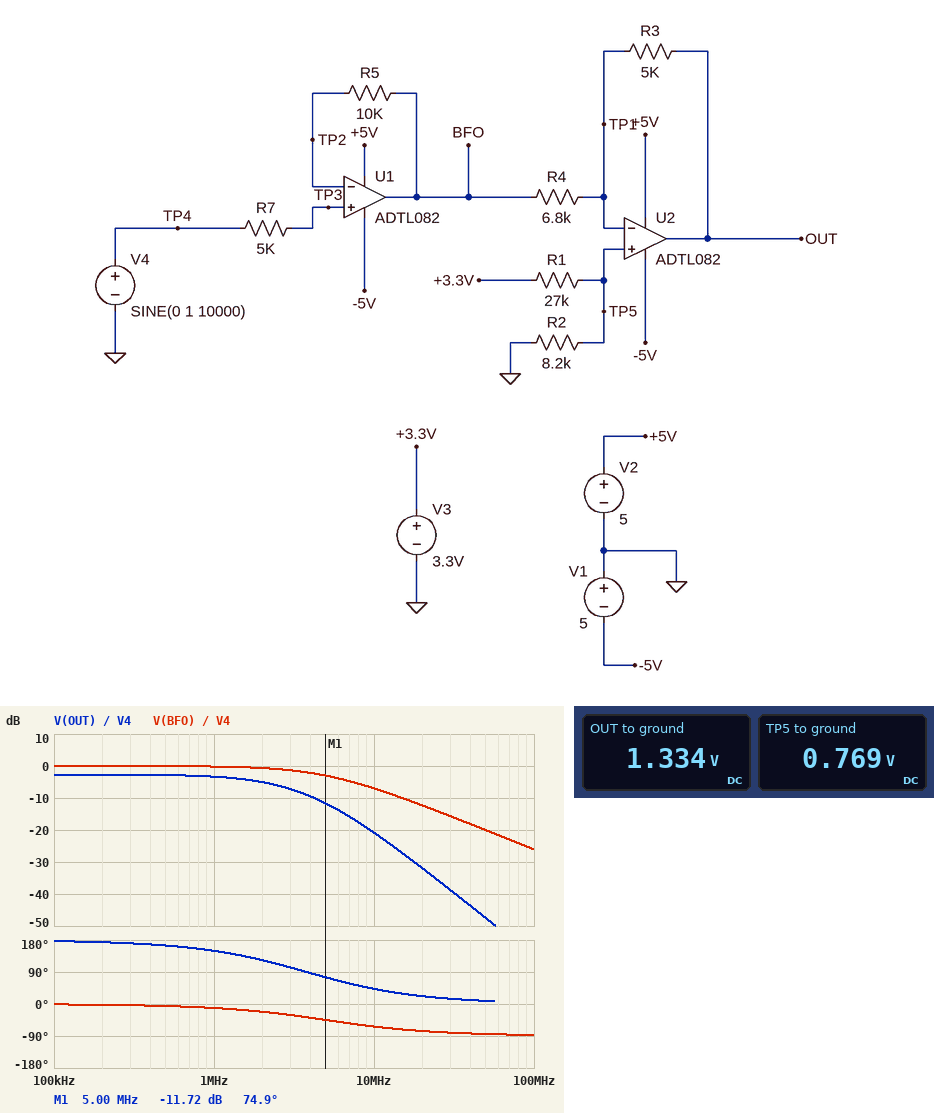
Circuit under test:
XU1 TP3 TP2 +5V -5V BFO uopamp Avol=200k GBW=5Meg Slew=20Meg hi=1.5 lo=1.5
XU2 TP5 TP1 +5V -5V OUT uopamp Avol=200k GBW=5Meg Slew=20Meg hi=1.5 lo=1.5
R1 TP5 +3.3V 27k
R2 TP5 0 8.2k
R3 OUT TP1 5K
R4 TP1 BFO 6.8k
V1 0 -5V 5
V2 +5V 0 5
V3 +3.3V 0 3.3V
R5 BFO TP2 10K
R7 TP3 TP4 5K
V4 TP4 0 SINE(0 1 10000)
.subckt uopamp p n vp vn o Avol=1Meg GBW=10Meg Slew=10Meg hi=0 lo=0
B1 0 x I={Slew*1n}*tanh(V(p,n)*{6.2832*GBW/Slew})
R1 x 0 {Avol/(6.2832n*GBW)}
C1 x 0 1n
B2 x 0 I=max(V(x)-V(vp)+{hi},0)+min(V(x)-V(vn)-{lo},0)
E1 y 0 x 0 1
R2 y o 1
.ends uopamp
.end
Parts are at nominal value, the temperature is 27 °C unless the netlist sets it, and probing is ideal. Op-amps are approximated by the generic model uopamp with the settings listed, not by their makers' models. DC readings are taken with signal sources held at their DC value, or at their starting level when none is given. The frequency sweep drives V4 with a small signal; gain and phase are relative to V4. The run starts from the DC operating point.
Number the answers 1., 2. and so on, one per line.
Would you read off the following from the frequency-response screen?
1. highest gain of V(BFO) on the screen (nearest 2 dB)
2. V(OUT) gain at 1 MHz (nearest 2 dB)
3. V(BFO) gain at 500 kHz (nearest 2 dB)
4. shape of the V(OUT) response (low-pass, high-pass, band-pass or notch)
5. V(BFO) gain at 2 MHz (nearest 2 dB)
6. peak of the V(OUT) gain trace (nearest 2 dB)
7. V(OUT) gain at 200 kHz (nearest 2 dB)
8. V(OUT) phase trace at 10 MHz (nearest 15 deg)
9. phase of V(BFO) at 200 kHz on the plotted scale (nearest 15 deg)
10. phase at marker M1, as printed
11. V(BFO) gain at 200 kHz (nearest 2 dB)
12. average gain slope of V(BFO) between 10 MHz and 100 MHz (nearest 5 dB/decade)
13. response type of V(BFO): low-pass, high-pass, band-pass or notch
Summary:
1. 0 dB
2. -4 dB
3. 0 dB
4. low-pass
5. 0 dB
6. -2 dB
7. -2 dB
8. 45 deg
9. 0 deg
10. 74.9 deg
11. 0 dB
12. -20 dB/decade
13. low-pass
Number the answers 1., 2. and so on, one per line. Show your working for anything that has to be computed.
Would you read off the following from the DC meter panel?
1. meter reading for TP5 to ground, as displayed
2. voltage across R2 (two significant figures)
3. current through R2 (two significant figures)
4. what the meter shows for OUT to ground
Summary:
1. 0.769 V
2. 769 mV = 770 mV
3. (769 mV) / 8.2 kΩ = 94 µA
4. 1.334 V
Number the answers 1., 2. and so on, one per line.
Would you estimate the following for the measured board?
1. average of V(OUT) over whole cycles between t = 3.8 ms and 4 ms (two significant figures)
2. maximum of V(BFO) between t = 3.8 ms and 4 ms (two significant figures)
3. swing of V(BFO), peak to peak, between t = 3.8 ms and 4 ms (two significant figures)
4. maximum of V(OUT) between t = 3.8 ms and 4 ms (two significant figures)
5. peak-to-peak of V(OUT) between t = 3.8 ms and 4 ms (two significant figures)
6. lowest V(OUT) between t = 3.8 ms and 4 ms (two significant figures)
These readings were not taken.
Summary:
1. 1.3 V
2. 1.0 V
3. 2.0 V
4. 2.1 V
5. 1.5 V
6. 600 mV
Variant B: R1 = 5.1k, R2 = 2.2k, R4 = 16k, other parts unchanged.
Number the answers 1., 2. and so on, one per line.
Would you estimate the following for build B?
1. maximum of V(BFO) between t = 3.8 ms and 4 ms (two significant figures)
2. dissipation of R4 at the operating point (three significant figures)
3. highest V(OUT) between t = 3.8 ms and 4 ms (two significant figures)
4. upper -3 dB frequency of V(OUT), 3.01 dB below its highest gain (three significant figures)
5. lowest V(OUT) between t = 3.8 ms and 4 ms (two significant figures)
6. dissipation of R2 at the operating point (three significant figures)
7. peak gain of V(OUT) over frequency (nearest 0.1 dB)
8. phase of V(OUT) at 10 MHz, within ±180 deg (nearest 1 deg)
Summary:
1. 1.0 V
2. 61.8 µW
3. 1.6 V
4. 2.77 MHz
5. 990 mV
6. 450 µW
7. -10.1 dB
8. 47 deg
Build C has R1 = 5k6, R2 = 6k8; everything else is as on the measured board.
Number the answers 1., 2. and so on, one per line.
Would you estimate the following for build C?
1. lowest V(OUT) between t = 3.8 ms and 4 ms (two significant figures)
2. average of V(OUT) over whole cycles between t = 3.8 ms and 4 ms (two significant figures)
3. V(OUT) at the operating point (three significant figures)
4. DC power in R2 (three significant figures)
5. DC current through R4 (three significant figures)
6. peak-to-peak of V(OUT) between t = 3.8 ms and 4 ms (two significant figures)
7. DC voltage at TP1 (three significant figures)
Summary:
1. 2.4 V
2. 3.1 V
3. 3.14 V
4. 482 µW
5. 266 µA
6. 1.1 V
7. 1.81 V
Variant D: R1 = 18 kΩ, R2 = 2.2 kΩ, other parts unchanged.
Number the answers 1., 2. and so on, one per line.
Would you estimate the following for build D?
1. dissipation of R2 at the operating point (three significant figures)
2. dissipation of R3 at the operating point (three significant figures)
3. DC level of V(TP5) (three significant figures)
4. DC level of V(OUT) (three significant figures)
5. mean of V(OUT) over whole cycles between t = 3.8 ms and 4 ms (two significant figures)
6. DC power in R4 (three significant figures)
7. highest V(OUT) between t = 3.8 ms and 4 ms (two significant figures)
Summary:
1. 58.7 µW
2. 14.0 µW
3. 359 mV
4. 624 mV
5. 620 mV
6. 19.0 µW
7. 1.4 V
